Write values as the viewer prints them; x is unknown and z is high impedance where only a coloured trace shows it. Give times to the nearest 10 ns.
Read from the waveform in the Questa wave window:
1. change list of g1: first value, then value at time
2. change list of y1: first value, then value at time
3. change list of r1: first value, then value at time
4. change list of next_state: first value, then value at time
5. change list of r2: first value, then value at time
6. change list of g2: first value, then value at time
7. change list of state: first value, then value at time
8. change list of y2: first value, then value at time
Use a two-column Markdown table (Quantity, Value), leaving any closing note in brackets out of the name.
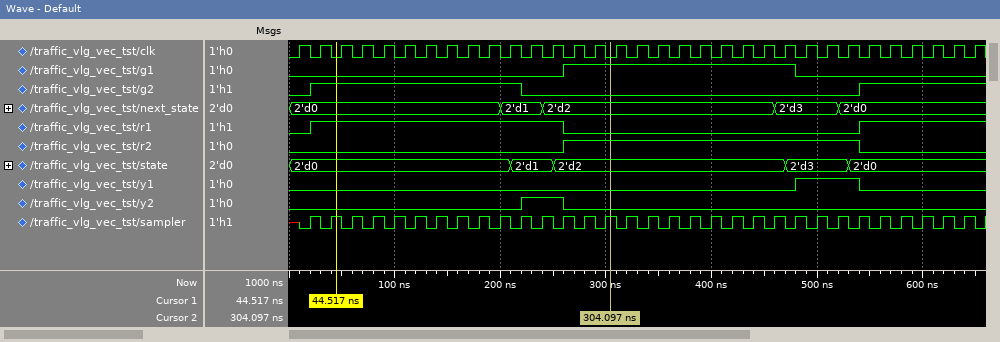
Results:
| Quantity | Value |
|---|---|
| change list of g1: first value, then value at time | 0, 1 at 260 ns, 0 at 480 ns |
| change list of y1: first value, then value at time | 0, 1 at 480 ns, 0 at 540 ns |
| change list of r1: first value, then value at time | 0, 1 at 20 ns, 0 at 260 ns, 1 at 540 ns |
| change list of next_state: first value, then value at time | 2'd0, 2'd1 at 200 ns, 2'd2 at 240 ns, 2'd3 at 460 ns, 2'd0 at 520 ns |
| change list of r2: first value, then value at time | 0, 1 at 260 ns, 0 at 540 ns |
| change list of g2: first value, then value at time | 0, 1 at 20 ns, 0 at 220 ns, 1 at 540 ns |
| change list of state: first value, then value at time | 2'd0, 2'd1 at 210 ns, 2'd2 at 250 ns, 2'd3 at 470 ns, 2'd0 at 530 ns |
| change list of y2: first value, then value at time | 0, 1 at 220 ns, 0 at 260 ns |
